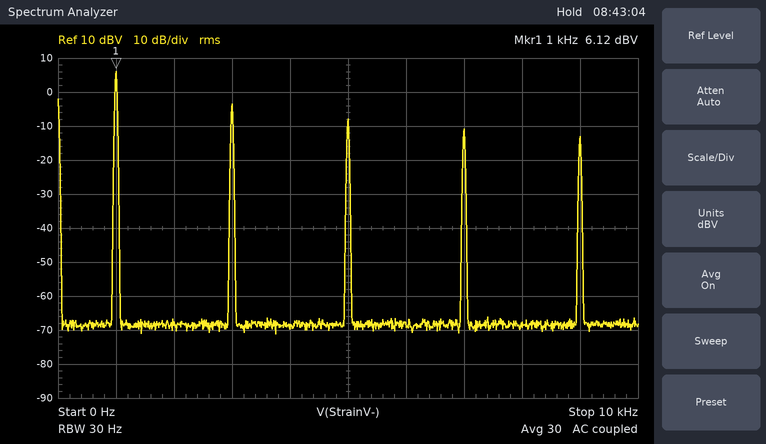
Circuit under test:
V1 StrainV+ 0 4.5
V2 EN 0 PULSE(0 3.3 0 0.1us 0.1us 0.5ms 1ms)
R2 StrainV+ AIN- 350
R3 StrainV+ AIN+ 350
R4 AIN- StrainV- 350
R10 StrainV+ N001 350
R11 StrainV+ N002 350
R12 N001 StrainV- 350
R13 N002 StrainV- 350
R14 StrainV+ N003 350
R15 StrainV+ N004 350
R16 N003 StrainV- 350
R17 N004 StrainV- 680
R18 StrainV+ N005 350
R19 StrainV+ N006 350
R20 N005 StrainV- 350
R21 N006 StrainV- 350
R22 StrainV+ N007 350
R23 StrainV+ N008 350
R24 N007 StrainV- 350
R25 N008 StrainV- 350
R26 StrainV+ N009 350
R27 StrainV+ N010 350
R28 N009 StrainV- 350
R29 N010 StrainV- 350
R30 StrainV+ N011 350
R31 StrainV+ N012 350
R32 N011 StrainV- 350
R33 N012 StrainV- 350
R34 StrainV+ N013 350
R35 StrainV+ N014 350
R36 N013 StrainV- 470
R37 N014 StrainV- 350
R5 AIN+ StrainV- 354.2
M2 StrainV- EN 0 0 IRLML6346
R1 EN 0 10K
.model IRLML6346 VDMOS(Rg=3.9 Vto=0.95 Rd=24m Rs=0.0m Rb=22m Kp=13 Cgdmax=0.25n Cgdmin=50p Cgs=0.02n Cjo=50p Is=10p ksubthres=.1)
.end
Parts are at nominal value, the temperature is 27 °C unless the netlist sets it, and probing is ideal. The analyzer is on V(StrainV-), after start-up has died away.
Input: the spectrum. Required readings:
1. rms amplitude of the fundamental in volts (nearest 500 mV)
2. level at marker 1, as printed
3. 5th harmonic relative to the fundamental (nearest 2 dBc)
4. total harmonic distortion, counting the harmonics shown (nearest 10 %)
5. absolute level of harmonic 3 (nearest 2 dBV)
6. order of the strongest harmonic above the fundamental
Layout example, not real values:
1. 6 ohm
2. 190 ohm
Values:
1. 2.0 V
2. 6.12 dBV
3. -14 dBc
4. 40 %
5. -4 dBV
6. 3
